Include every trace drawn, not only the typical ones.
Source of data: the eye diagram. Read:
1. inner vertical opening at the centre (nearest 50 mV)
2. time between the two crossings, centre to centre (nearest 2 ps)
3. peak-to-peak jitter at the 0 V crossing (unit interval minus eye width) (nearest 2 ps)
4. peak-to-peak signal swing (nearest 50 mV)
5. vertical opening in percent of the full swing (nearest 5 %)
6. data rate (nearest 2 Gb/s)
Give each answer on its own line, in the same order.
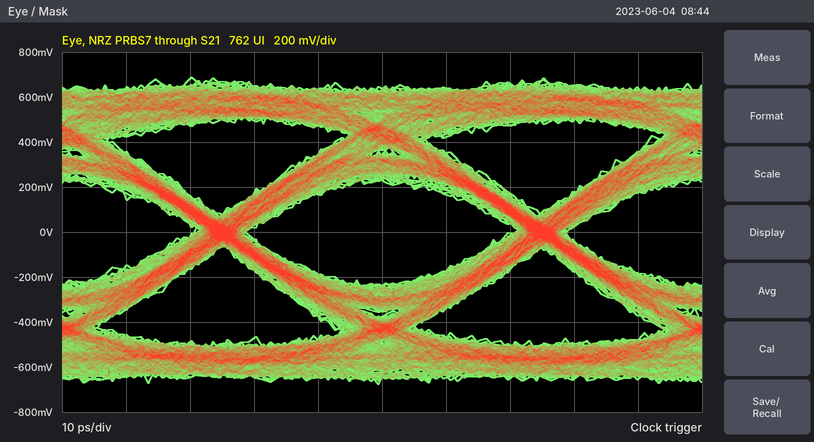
450 mV
50 ps
8 ps
1.35 V
35 %
20 Gb/s
